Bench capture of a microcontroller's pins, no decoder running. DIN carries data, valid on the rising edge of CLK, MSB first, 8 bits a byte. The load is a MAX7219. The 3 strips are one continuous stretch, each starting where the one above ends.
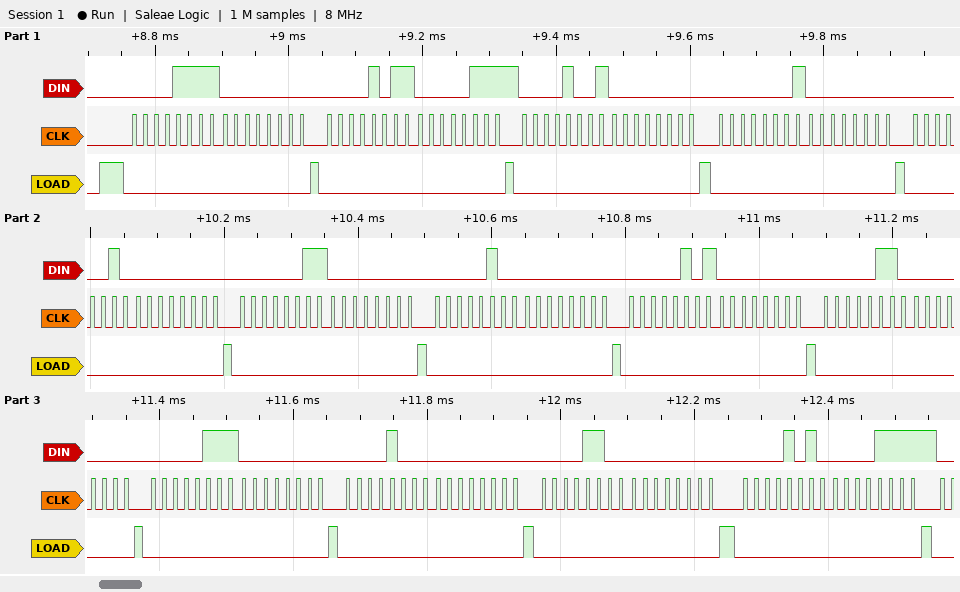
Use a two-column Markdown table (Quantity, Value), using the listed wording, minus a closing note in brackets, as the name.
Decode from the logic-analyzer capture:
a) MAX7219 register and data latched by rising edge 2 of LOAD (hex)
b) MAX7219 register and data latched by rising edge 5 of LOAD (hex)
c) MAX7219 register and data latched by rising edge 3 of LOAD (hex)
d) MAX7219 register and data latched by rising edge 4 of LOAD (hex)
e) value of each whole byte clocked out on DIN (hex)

| Quantity | Value |
|---|---|
| MAX7219 register and data latched by rising edge 2 of LOAD | register 0xF, data 0x00 |
| MAX7219 register and data latched by rising edge 5 of LOAD | register 0x1, data 0x00 |
| MAX7219 register and data latched by rising edge 3 of LOAD | register 0xB, data 0x07 |
| MAX7219 register and data latched by rising edge 4 of LOAD | register 0x9, data 0x00 |
| value of each whole byte clocked out on DIN | 0x0F 0x00 0x0B 0x07 0x09 0x00 0x01 0x00 0x02 0x00 0x03 0x00 0x04 0x00 0x05 0x00 0x06 0x00 0x07 0x00 0x08 0x00 0x0C 0x00 0x0A 0x0F |
